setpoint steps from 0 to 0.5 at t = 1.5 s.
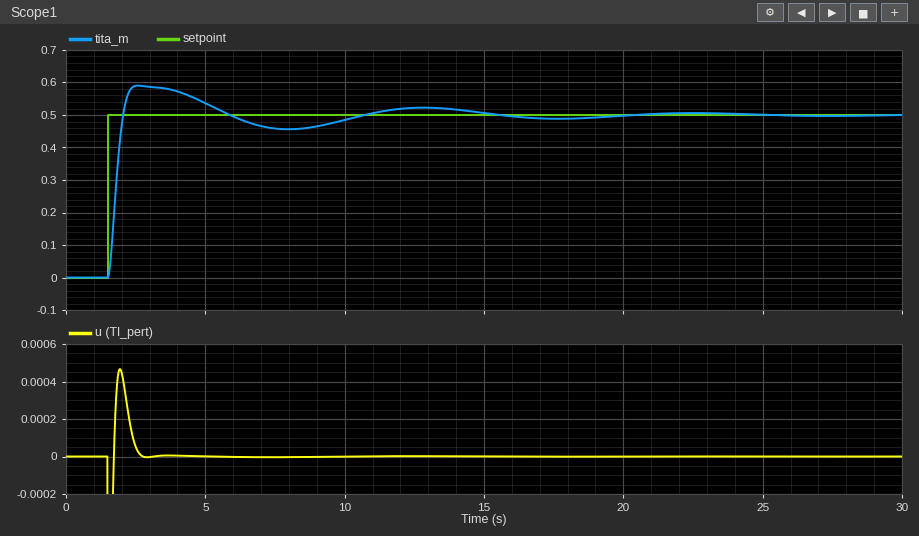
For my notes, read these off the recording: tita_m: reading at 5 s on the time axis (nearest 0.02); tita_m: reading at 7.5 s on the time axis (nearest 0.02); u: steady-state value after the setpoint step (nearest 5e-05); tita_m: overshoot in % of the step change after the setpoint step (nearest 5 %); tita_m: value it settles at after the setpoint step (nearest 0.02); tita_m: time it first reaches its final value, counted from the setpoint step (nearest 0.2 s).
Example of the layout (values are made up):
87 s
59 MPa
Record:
0.54
0.46
0.00000
20 %
0.50
0.6 s
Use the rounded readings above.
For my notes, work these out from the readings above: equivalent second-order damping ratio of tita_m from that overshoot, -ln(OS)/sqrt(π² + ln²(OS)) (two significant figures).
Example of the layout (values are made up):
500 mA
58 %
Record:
0.46
